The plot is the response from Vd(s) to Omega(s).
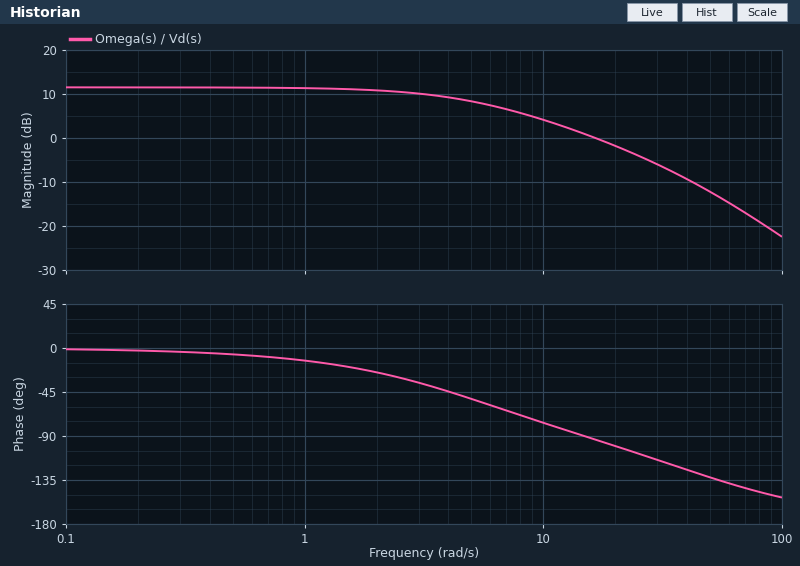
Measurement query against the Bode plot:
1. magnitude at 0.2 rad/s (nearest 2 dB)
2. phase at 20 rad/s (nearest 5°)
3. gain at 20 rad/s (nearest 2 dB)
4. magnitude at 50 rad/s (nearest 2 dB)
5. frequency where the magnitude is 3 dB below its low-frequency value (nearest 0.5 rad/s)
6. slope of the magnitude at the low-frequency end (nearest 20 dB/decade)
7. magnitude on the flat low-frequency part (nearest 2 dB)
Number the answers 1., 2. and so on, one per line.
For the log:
1. 12 dB
2. -100°
3. -2 dB
4. -12 dB
5. 5.0 rad/s
6. 0 dB/decade
7. 12 dB
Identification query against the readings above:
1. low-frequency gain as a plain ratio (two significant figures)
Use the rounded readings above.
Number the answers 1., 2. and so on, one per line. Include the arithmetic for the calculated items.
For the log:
1. 10^(12 / 20) = 4.0
